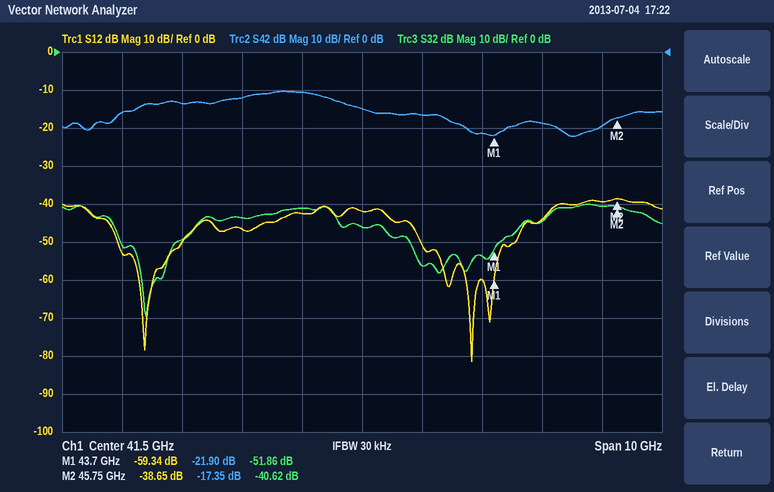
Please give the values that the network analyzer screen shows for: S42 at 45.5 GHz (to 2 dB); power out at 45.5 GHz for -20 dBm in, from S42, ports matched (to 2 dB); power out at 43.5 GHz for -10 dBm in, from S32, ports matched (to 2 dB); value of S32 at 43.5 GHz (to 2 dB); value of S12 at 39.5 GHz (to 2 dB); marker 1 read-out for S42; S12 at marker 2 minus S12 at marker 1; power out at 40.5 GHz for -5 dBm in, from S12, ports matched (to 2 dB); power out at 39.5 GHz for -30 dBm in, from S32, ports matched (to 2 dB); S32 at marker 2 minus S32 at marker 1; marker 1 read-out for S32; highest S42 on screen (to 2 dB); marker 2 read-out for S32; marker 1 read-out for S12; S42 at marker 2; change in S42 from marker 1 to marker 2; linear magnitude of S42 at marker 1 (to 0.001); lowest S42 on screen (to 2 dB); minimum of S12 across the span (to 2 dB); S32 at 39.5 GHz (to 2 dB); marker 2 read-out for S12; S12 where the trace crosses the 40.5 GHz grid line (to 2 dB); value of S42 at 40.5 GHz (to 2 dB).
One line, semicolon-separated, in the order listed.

-20 dB; -40 dBm; -64 dBm; -54 dB; -46 dB; -21.90 dB; 20.69 dB; -48 dBm; -74 dBm; 11.24 dB; -51.86 dB; -10 dB; -40.62 dB; -59.34 dB; -17.35 dB; 4.55 dB; 0.080; -22 dB; -82 dB; -44 dB; -38.65 dB; -42 dB; -10 dB
